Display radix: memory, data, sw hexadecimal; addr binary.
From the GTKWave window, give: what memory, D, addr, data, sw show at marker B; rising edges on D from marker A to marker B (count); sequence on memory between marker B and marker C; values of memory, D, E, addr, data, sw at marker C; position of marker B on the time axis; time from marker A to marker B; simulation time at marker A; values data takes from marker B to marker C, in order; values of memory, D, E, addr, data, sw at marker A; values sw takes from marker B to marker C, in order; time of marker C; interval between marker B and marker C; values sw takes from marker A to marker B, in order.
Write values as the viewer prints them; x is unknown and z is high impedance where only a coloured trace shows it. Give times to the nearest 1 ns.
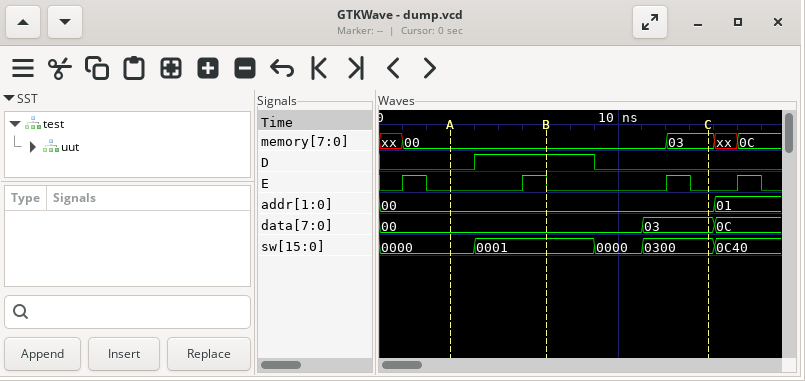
memory=00, D=1, addr=00, data=00, sw=0001
1
00, 03
memory=03, D=0, E=0, addr=00, data=03, sw=0300
7 ns
4 ns
3 ns
00, 03
memory=00, D=0, E=0, addr=00, data=00, sw=0000
0001, 0000, 0300
14 ns
7 ns
0000, 0001
